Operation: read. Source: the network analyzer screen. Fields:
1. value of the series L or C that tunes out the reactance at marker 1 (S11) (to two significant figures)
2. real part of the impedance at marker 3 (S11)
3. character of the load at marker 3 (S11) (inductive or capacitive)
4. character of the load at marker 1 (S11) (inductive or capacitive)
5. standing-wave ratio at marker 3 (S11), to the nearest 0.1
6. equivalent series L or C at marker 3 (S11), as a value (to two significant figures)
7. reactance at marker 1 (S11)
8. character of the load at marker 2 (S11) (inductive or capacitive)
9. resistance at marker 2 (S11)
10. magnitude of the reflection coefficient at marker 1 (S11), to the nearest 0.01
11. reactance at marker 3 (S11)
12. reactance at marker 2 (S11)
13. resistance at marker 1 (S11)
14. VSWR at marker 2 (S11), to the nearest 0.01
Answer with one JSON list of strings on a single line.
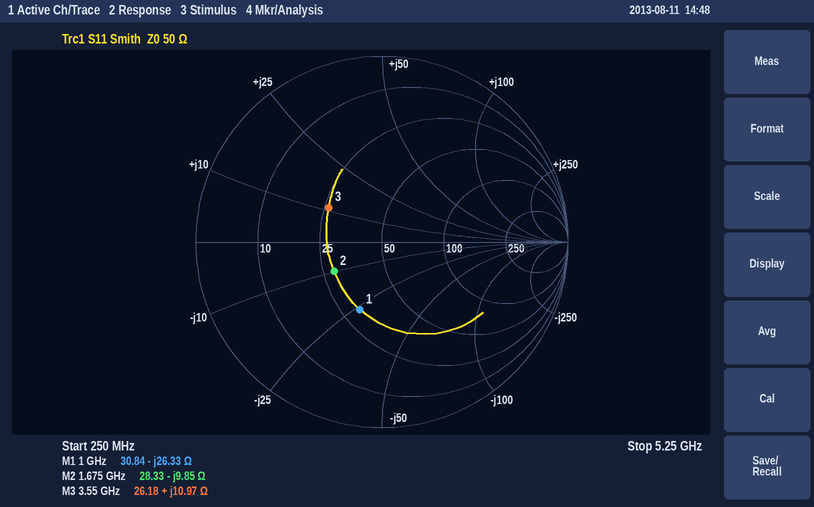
["4.2 nH", "26.18 Ω", "inductive", "capacitive", "2.0", "490 pH", "-26.33 Ω", "capacitive", "28.33 Ω", "0.38", "+10.97 Ω", "-9.85 Ω", "30.84 Ω", "1.86"]
